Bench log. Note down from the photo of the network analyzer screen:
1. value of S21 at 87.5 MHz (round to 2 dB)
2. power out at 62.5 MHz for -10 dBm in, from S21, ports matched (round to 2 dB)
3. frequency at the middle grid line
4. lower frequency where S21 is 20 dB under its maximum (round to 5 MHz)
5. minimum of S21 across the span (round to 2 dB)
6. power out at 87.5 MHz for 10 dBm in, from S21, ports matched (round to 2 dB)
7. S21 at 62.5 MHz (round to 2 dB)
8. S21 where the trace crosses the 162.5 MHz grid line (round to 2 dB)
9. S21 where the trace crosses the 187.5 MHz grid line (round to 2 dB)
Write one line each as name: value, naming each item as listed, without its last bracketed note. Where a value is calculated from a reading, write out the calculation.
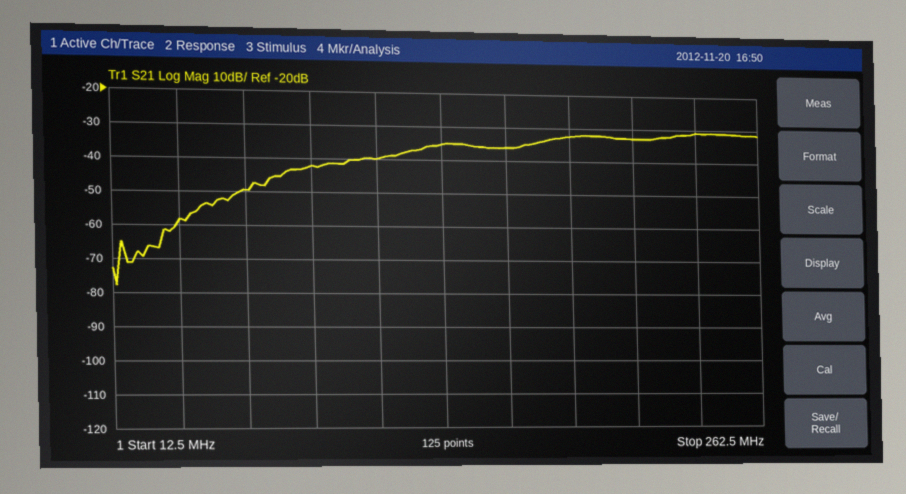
value of S21 at 87.5 MHz: -42 dB
power out at 62.5 MHz for -10 dBm in, from S21, ports matched: -10 dBm + (-50 dB) = -60 dBm
frequency at the middle grid line: 137.5 MHz
lower frequency where S21 is 20 dB under its maximum: 60 MHz
minimum of S21 across the span: -78 dB
power out at 87.5 MHz for 10 dBm in, from S21, ports matched: 10 dBm + (-42 dB) = -32 dBm
S21 at 62.5 MHz: -50 dB
S21 where the trace crosses the 162.5 MHz grid line: -36 dB
S21 where the trace crosses the 187.5 MHz grid line: -32 dB
